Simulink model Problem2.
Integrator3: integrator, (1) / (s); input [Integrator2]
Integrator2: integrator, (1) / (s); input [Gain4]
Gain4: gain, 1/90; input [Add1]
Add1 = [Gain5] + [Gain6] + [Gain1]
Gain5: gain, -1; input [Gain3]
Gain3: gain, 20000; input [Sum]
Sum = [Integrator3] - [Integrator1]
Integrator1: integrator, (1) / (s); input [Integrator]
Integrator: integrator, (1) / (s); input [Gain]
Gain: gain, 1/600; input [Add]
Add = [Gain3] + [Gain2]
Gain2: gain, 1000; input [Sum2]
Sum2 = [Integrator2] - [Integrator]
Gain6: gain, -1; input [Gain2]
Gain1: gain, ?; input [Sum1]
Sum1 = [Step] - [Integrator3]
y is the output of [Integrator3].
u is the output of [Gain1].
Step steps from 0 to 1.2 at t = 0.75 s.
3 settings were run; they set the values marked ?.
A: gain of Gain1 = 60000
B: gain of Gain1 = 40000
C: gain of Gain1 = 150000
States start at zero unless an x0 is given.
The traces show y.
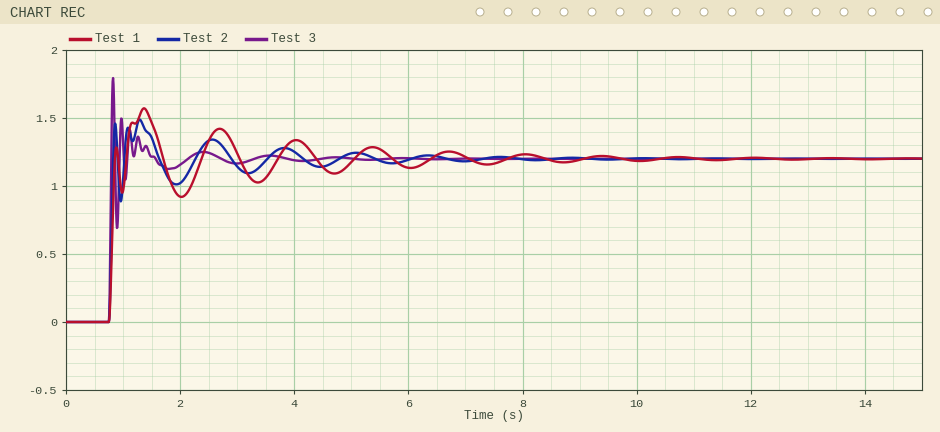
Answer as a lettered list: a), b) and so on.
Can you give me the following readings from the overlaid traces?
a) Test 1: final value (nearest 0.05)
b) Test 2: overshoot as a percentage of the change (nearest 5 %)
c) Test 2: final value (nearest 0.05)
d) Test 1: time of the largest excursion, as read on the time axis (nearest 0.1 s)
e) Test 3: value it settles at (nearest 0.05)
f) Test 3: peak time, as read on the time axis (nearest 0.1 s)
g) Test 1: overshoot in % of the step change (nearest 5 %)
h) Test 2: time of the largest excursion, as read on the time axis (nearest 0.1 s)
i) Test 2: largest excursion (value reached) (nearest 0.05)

a) 1.20
b) 25 %
c) 1.20
d) 1.4 s
e) 1.20
f) 0.8 s
g) 30 %
h) 1.3 s
i) 1.50
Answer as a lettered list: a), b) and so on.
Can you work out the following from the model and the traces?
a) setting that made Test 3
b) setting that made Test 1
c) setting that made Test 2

a) C
b) B
c) A
